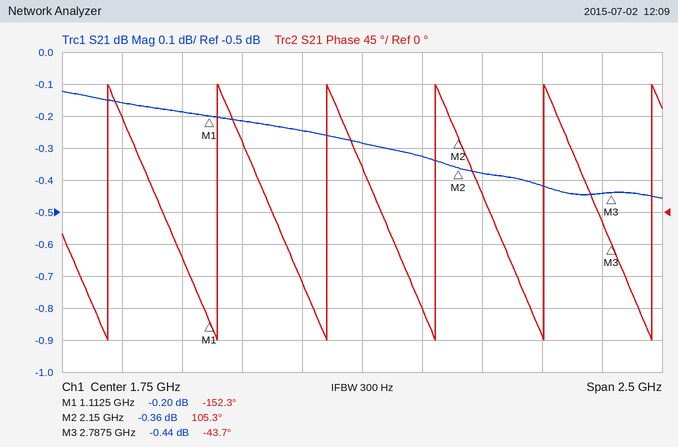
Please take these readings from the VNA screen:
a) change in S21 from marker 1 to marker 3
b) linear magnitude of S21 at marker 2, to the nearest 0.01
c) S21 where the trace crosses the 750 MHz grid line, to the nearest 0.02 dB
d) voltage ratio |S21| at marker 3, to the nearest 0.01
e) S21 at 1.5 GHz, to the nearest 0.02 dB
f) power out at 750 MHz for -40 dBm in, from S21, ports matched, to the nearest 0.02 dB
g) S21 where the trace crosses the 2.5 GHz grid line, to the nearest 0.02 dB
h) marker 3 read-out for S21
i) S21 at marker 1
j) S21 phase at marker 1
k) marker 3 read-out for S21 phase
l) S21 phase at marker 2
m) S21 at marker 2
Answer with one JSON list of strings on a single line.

["-0.24 dB", "0.96", "-0.16 dB", "0.95", "-0.24 dB", "-40.16 dBm", "-0.42 dB", "-0.44 dB", "-0.20 dB", "-152.3°", "-43.7°", "105.3°", "-0.36 dB"]
